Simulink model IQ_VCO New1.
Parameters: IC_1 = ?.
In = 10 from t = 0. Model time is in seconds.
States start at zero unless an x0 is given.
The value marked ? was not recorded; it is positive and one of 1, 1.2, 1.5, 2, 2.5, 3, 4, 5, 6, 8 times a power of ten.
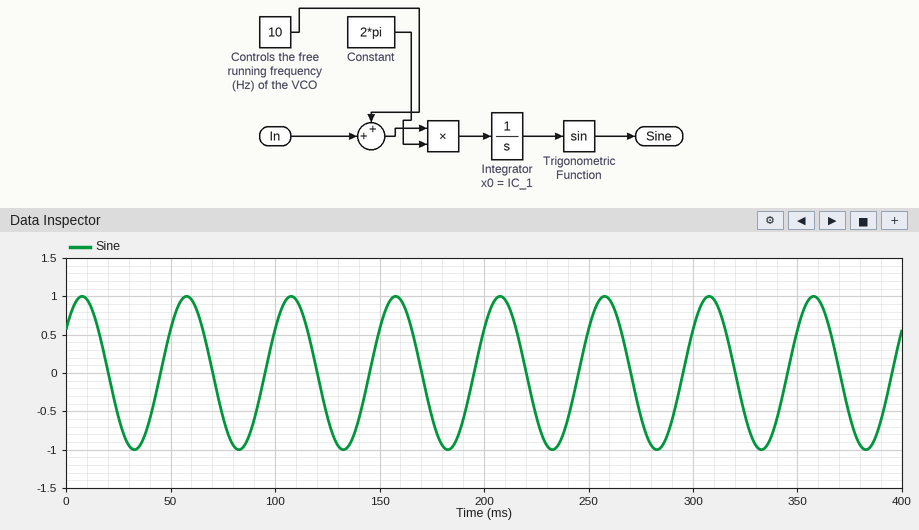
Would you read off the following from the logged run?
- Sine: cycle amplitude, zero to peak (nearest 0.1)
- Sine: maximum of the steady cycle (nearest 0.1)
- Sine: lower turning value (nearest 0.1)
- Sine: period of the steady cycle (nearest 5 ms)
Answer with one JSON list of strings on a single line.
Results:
["1.0", "1.0", "-1.0", "50 ms"]
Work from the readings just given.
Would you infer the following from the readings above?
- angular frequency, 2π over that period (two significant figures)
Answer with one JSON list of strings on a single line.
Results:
["0.13 rad/ms"]
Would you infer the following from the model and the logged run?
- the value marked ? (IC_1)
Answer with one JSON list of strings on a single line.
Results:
["0.6"]
